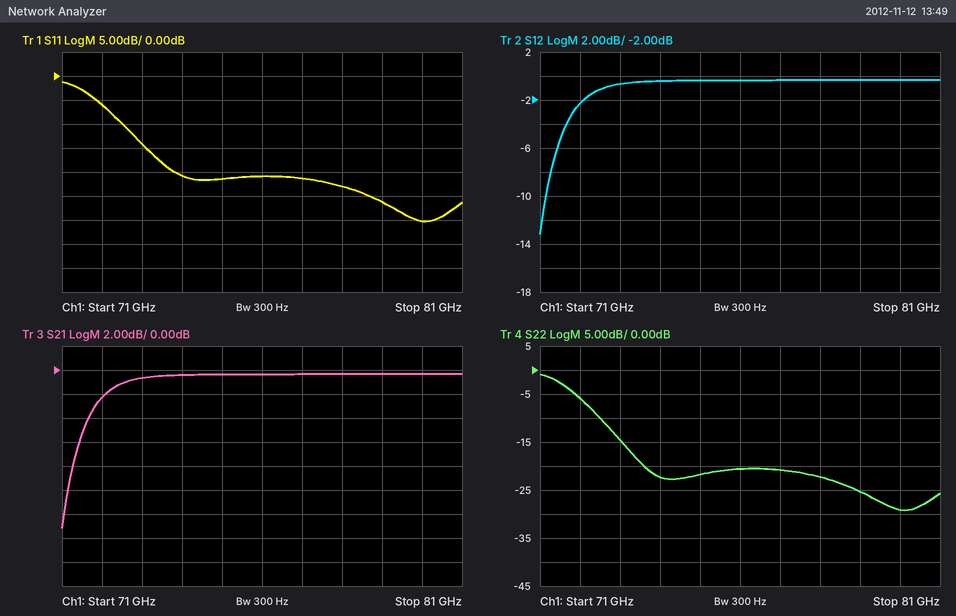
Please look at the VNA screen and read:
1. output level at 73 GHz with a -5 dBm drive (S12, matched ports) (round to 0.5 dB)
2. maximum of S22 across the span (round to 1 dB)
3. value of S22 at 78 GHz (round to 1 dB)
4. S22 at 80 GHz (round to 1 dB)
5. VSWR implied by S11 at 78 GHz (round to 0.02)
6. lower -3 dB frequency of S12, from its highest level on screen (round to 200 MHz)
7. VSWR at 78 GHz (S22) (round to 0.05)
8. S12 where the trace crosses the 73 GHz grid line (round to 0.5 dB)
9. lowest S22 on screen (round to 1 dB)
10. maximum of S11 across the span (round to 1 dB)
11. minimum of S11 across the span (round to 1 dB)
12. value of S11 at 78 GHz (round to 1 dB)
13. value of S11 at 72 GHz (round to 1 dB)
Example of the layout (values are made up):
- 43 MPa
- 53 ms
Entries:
- -5.5 dBm
- -1 dB
- -22 dB
- -29 dB
- 1.16
- 71.8 GHz
- 1.15
- -0.5 dB
- -29 dB
- -1 dB
- -30 dB
- -23 dB
- -6 dB
